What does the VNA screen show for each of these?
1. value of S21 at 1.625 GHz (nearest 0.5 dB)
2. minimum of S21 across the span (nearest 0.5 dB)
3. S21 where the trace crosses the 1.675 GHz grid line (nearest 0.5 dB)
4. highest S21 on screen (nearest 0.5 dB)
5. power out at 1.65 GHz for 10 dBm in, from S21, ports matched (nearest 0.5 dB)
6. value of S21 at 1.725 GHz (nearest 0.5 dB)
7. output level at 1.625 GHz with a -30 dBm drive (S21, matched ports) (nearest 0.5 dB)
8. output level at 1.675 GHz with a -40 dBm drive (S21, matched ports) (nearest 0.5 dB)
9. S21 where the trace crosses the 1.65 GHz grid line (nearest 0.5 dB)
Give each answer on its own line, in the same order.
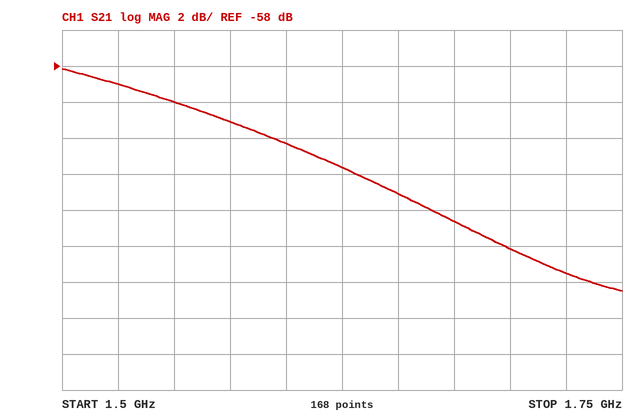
-63.5 dB
-70.5 dB
-66.5 dB
-58.0 dB
-55.0 dBm
-69.5 dB
-93.5 dBm
-106.5 dBm
-65.0 dB
